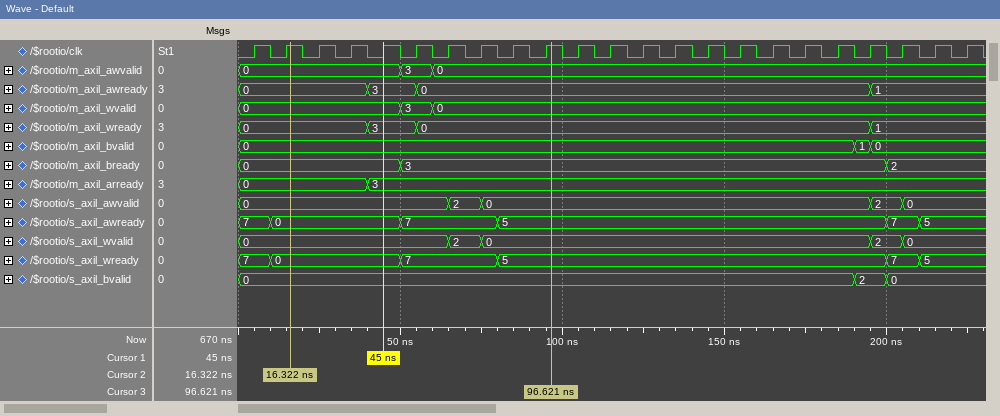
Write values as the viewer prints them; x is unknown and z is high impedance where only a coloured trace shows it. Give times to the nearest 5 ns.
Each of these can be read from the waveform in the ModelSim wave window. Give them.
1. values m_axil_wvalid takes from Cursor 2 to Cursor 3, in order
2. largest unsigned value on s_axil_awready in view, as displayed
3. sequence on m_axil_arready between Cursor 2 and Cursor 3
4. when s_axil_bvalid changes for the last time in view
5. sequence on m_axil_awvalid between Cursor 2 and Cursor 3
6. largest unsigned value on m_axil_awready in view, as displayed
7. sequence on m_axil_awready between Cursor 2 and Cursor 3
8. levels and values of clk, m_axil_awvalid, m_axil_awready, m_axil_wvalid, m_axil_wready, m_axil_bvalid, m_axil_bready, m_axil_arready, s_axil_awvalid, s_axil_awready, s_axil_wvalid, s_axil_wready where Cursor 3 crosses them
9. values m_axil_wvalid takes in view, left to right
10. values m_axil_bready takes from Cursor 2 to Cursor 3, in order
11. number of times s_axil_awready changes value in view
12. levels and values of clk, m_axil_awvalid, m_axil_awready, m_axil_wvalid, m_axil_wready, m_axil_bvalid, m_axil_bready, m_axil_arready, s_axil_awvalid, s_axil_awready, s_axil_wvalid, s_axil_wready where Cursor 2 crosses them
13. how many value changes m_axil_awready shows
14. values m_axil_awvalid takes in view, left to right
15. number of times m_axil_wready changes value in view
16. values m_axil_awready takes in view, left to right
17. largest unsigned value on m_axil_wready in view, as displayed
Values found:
0, 3, 0
7
0, 3
200 ns
0, 3, 0
3
0, 3, 0
clk=1, m_axil_awvalid=0, m_axil_awready=0, m_axil_wvalid=0, m_axil_wready=0, m_axil_bvalid=0, m_axil_bready=3, m_axil_arready=3, s_axil_awvalid=0, s_axil_awready=5, s_axil_wvalid=0, s_axil_wready=5
0, 3, 0
0, 3
5
clk=1, m_axil_awvalid=0, m_axil_awready=0, m_axil_wvalid=0, m_axil_wready=0, m_axil_bvalid=0, m_axil_bready=0, m_axil_arready=0, s_axil_awvalid=0, s_axil_awready=0, s_axil_wvalid=0, s_axil_wready=0
3
0, 3, 0
3
0, 3, 0, 1
3
